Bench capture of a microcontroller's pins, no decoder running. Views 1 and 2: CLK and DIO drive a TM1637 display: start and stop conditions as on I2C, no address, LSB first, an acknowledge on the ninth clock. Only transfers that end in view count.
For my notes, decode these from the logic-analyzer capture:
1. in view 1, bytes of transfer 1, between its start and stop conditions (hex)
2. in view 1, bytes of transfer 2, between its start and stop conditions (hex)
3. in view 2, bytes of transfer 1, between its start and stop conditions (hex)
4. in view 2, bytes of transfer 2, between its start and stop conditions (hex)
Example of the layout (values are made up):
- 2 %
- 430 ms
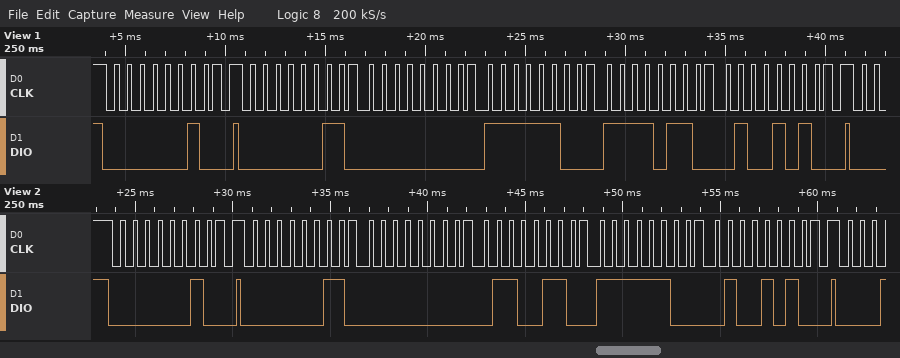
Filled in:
- 40
- C0 00 3F 6F 52
- 40
- C0 00 66 3F 52
